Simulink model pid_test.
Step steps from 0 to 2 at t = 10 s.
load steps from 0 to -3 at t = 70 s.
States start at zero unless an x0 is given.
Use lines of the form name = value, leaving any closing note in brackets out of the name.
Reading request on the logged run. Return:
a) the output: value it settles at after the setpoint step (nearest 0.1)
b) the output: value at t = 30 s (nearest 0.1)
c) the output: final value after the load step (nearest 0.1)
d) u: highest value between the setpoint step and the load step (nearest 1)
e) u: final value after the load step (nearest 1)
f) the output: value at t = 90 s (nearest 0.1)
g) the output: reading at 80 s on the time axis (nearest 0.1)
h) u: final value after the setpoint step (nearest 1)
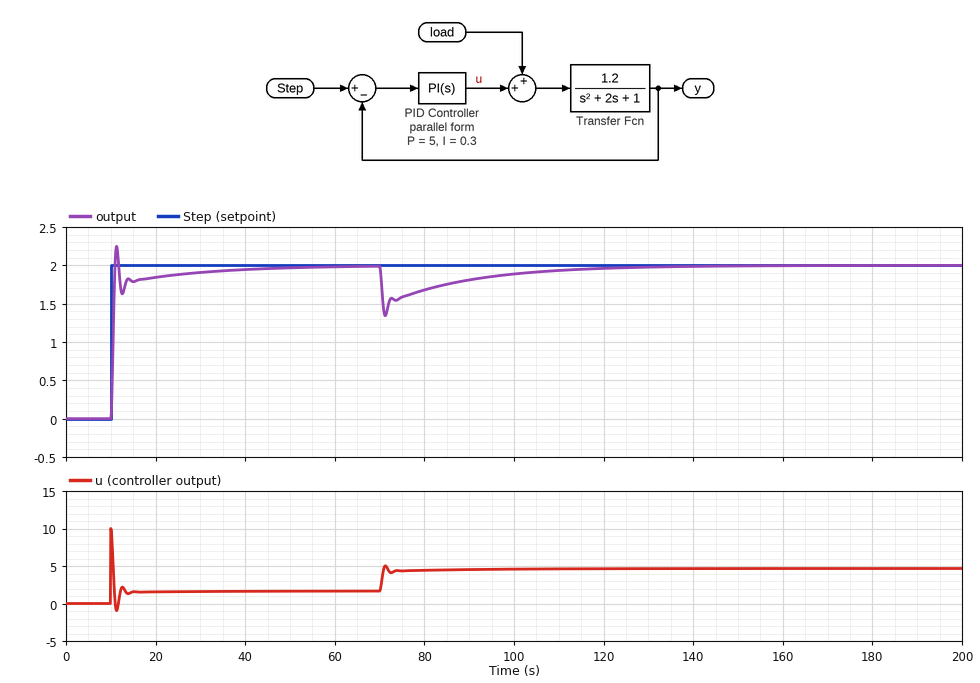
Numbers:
the output: value it settles at after the setpoint step = 2.0
the output: value at t = 30 s = 1.9
the output: final value after the load step = 2.0
u: highest value between the setpoint step and the load step = 10
u: final value after the load step = 5
the output: value at t = 90 s = 1.8
the output: reading at 80 s on the time axis = 1.7
u: final value after the setpoint step = 2
